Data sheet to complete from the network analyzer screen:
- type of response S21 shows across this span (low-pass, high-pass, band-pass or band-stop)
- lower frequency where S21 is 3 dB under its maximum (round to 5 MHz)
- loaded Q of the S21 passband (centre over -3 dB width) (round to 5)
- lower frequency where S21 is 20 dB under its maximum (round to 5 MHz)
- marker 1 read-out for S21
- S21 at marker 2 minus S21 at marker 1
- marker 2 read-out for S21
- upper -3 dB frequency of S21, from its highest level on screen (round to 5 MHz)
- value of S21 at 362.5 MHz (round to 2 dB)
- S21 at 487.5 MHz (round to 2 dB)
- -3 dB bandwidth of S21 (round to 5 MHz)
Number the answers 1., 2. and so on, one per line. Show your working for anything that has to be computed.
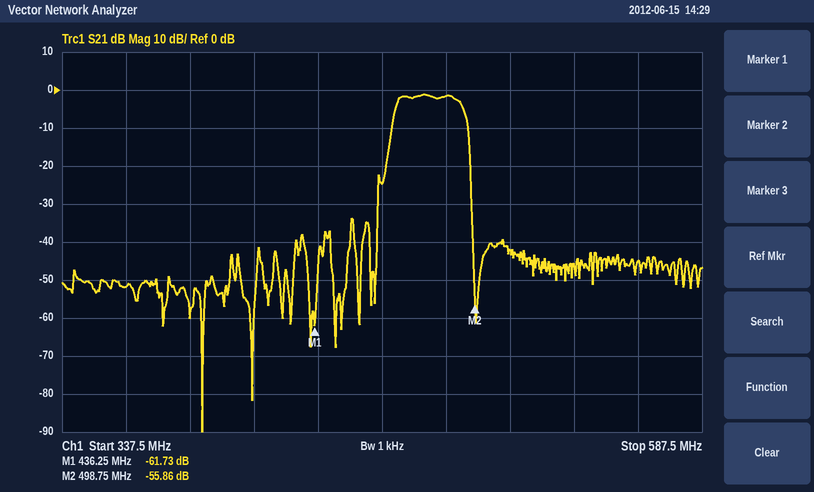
1. band-pass
2. 470 MHz
3. 482.5 MHz / 25 MHz ≈ 19.3, so 20 to the nearest 5
4. 465 MHz
5. -61.73 dB
6. -55.86 − (-61.73) = 5.87 dB
7. -55.86 dB
8. 495 MHz
9. -52 dB
10. -2 dB
11. 495 MHz − 470 MHz = 25 MHz
